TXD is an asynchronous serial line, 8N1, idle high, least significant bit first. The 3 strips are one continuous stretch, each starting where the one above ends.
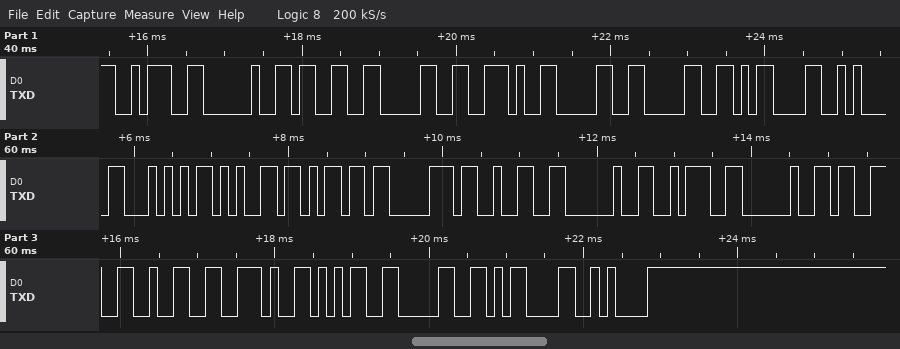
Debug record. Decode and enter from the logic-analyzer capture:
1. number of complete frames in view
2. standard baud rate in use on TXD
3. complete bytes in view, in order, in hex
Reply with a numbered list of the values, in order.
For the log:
1. 24
2. 9600 baud
3. 3A 20 33 30 2E 30 30 0D 0A 54 65 6D 70 32 20 3A 20 33 32 2E 35 30 0D 0A
